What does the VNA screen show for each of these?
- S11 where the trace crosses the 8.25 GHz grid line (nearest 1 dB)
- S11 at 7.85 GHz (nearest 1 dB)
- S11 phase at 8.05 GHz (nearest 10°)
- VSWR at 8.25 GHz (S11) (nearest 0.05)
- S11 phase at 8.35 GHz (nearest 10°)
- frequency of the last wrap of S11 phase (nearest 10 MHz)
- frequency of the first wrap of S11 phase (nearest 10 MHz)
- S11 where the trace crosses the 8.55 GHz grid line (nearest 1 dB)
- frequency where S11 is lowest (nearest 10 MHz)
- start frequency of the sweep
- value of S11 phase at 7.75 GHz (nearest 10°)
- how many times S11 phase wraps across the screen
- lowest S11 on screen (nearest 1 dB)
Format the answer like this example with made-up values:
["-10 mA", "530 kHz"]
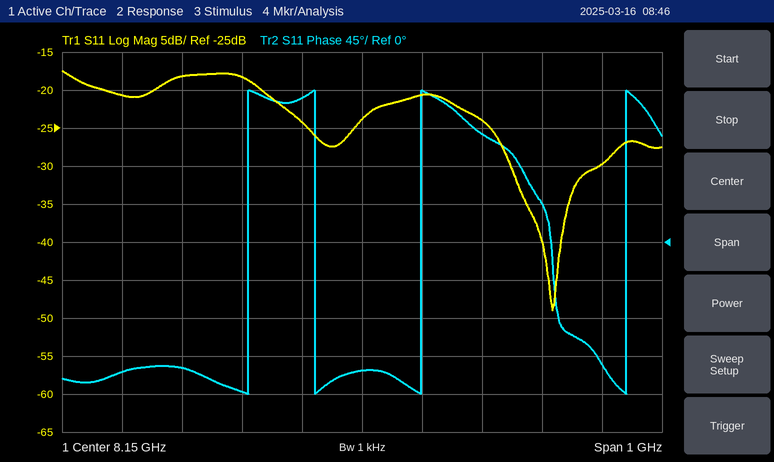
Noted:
["-21 dB", "-18 dB", "170°", "1.20", "130°", "8.59 GHz", "7.96 GHz", "-30 dB", "8.47 GHz", "7.65 GHz", "-150°", "4", "-49 dB"]
